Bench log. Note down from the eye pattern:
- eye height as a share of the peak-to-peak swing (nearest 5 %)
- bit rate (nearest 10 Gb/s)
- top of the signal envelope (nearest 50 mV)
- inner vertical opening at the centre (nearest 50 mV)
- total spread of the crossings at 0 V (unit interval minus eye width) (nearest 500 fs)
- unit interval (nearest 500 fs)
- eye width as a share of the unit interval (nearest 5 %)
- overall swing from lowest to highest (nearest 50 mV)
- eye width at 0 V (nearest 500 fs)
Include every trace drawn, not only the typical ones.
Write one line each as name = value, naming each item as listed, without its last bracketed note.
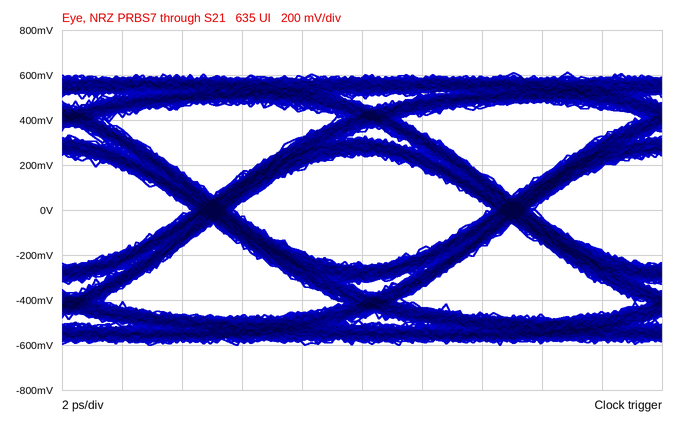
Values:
eye height as a share of the peak-to-peak swing = 40 %
bit rate = 100 Gb/s
top of the signal envelope = 600 mV
inner vertical opening at the centre = 500 mV
total spread of the crossings at 0 V (unit interval minus eye width) = 1.5 ps
unit interval = 10.0 ps
eye width as a share of the unit interval = 85 %
overall swing from lowest to highest = 1.20 V
eye width at 0 V = 8.5 ps
